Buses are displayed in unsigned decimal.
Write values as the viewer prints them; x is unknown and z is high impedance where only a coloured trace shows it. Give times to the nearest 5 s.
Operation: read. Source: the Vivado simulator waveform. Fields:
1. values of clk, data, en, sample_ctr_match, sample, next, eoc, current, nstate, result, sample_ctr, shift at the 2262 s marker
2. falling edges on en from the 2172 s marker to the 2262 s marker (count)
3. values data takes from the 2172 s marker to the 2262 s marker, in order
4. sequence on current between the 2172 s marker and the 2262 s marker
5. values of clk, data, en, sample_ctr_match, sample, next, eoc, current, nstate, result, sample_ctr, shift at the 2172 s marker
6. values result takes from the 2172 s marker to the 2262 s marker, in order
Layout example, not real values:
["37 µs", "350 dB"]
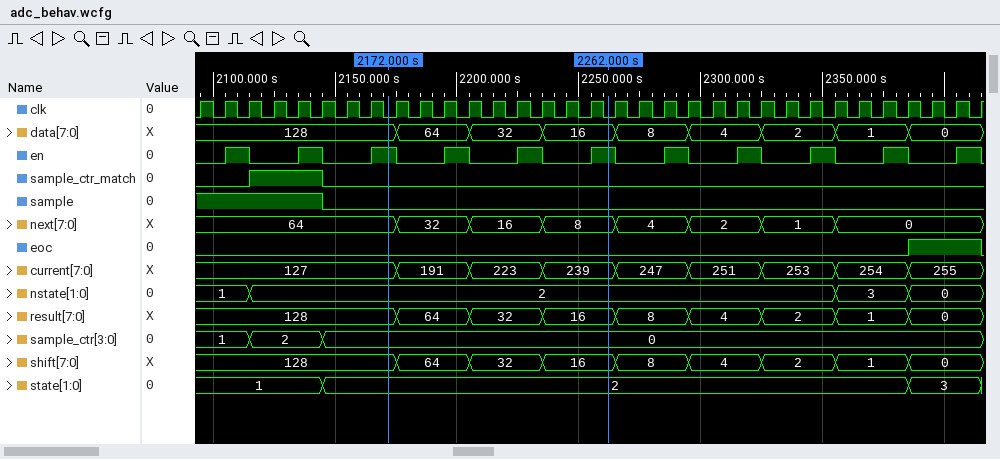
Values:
["clk=0, data=16, en=1, sample_ctr_match=0, sample=0, next=8, eoc=0, current=239, nstate=2, result=16, sample_ctr=0, shift=16", "3", "128, 64, 32, 16", "127, 191, 223, 239", "clk=0, data=128, en=1, sample_ctr_match=0, sample=0, next=64, eoc=0, current=127, nstate=2, result=128, sample_ctr=0, shift=128", "128, 64, 32, 16"]
